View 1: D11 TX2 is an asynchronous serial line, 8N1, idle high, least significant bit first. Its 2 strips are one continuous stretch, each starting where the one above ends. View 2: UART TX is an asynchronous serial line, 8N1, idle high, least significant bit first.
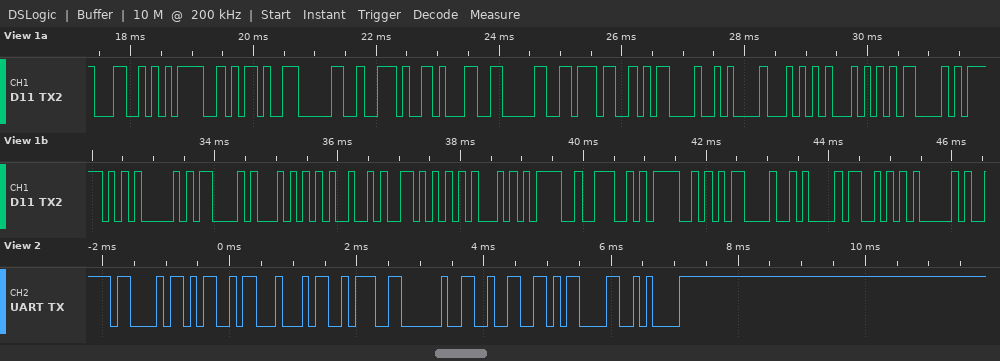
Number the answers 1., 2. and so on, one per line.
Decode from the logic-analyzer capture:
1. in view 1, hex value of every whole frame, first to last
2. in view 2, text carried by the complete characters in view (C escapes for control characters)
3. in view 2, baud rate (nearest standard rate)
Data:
1. 4C 3D 2D 30 2E 31 30 37 0D 0A 54 54 43 5F 41 43 54 49 56 45 3D 4E 4F 0D 0A 53 41
2. "CMD: 2\r\n"
3. 9600 baud
